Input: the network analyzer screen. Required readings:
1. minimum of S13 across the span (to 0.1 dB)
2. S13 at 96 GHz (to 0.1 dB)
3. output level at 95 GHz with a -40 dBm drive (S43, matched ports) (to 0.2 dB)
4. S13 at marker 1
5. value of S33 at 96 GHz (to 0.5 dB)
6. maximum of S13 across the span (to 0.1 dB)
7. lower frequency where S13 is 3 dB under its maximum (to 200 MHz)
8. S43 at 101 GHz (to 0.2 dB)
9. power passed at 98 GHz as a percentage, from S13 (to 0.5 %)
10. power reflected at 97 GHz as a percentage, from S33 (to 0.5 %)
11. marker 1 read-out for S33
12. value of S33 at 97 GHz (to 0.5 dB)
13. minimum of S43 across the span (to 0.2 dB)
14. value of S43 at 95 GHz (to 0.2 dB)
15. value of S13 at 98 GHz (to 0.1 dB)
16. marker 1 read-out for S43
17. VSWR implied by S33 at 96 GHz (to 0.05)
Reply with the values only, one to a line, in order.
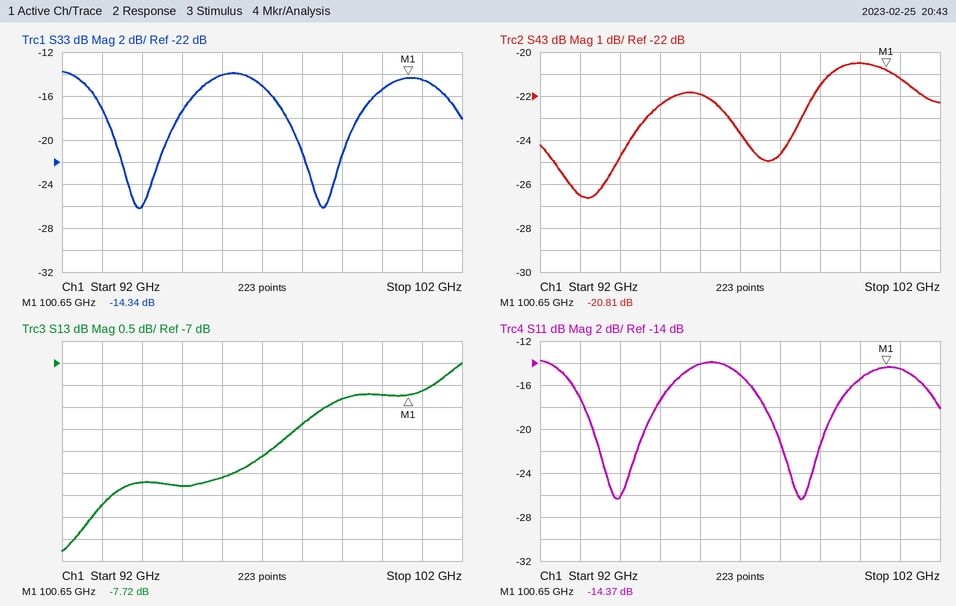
-11.3 dB
-9.6 dB
-62.4 dBm
-7.72 dB
-14.0 dB
-7.0 dB
93.2 GHz
-21.2 dB
14.5 %
3.0 %
-14.34 dB
-15.0 dB
-26.6 dB
-22.4 dB
-8.4 dB
-20.81 dB
1.50
